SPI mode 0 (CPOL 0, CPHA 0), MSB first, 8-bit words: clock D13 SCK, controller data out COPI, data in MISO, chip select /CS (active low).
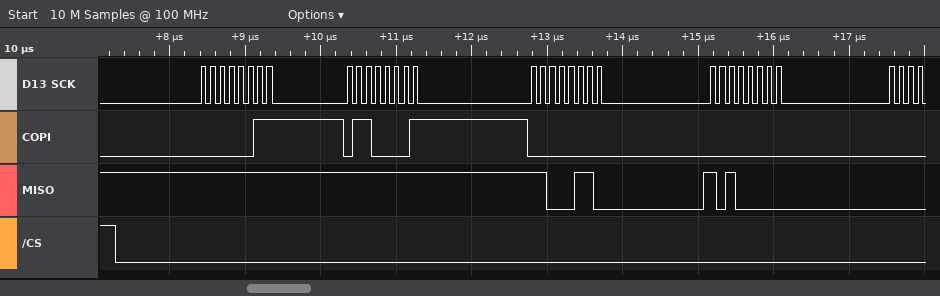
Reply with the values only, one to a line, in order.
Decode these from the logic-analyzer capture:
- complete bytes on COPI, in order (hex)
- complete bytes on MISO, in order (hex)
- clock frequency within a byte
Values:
03 61 00 00
FF FF C6 A0
8 MHz
